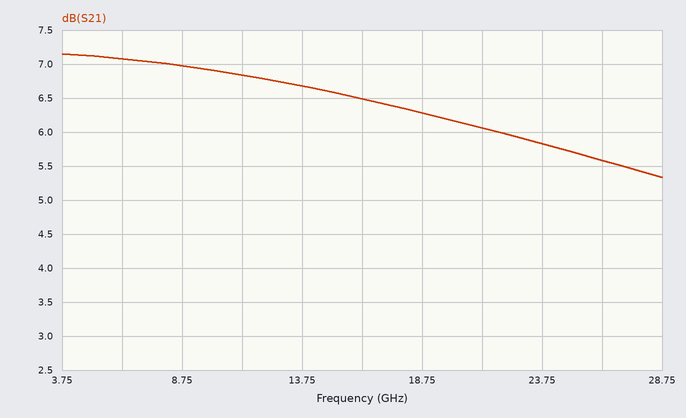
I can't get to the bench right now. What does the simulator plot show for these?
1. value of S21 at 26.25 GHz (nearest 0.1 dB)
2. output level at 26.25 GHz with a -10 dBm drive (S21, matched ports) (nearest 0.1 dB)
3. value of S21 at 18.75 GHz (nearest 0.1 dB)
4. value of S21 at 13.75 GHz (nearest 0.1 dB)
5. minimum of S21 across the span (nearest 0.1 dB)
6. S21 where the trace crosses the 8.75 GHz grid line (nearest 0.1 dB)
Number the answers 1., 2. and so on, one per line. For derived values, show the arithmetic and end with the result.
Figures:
1. 5.6 dB
2. -10 dBm + (5.6 dB) = -4.4 dBm
3. 6.3 dB
4. 6.7 dB
5. 5.3 dB
6. 7.0 dB
